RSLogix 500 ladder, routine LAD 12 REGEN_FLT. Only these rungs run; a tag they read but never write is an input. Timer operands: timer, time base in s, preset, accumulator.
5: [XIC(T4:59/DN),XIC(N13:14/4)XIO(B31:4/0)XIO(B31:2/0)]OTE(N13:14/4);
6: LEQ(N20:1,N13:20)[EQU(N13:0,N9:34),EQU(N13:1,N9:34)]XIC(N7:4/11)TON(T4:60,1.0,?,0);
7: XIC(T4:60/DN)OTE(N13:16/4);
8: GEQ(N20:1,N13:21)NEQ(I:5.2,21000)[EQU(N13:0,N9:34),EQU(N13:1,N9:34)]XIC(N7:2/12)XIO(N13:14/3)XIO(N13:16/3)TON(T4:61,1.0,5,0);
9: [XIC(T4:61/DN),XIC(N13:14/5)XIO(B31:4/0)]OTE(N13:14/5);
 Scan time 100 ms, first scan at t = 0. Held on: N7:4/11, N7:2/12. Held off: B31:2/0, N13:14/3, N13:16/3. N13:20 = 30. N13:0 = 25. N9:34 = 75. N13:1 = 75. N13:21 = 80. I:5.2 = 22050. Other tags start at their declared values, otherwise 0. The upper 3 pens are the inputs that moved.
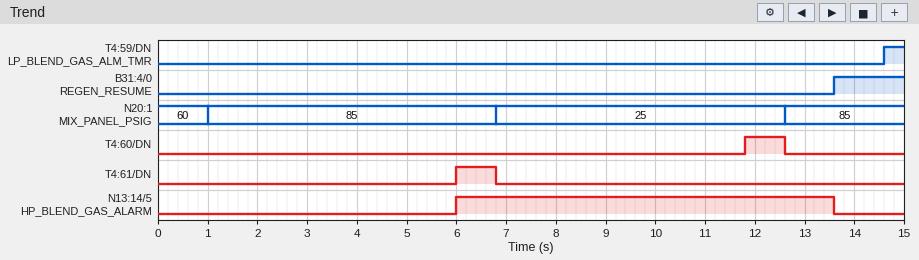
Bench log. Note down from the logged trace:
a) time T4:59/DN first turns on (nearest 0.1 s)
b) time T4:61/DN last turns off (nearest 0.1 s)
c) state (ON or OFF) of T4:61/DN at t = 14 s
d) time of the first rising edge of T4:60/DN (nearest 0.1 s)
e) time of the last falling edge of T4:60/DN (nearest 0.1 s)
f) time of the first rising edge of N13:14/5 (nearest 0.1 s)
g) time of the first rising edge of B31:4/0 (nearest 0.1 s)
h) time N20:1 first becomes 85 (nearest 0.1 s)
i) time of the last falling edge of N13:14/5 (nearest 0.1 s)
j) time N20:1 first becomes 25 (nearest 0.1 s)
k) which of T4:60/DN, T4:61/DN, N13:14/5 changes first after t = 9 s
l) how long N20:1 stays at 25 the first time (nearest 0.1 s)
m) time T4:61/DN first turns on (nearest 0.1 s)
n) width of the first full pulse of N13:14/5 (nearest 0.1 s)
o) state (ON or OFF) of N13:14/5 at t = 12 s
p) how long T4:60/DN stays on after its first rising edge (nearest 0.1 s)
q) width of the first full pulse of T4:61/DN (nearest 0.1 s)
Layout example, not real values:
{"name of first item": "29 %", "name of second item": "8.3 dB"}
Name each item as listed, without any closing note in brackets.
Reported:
{"time T4:59/DN first turns on": "14.6 s", "time T4:61/DN last turns off": "6.8 s", "state (ON or OFF) of T4:61/DN at t = 14 s": "OFF", "time of the first rising edge of T4:60/DN": "11.8 s", "time of the last falling edge of T4:60/DN": "12.6 s", "time of the first rising edge of N13:14/5": "6.0 s", "time of the first rising edge of B31:4/0": "13.6 s", "time N20:1 first becomes 85": "1.0 s", "time of the last falling edge of N13:14/5": "13.6 s", "time N20:1 first becomes 25": "6.8 s", "which of T4:60/DN, T4:61/DN, N13:14/5 changes first after t = 9 s": "T4:60/DN", "how long N20:1 stays at 25 the first time": "5.8 s", "time T4:61/DN first turns on": "6.0 s", "width of the first full pulse of N13:14/5": "7.6 s", "state (ON or OFF) of N13:14/5 at t = 12 s": "ON", "how long T4:60/DN stays on after its first rising edge": "0.8 s", "width of the first full pulse of T4:61/DN": "0.8 s"}
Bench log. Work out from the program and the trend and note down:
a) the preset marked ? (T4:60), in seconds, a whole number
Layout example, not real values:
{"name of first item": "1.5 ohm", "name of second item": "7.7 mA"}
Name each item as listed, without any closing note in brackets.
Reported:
{"the preset marked ? (T4:60), in seconds, a whole number": "5 s"}
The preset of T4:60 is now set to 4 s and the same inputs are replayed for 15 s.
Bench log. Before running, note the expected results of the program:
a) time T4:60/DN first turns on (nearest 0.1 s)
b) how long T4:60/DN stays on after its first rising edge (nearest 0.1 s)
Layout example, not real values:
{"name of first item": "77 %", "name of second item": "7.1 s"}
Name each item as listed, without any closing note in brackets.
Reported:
{"time T4:60/DN first turns on": "10.8 s", "how long T4:60/DN stays on after its first rising edge": "1.8 s"}
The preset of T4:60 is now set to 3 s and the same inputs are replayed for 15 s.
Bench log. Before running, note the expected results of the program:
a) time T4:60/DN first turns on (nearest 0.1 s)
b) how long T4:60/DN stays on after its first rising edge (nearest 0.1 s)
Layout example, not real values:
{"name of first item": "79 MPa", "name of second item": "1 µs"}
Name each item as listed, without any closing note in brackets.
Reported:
{"time T4:60/DN first turns on": "9.8 s", "how long T4:60/DN stays on after its first rising edge": "2.8 s"}
